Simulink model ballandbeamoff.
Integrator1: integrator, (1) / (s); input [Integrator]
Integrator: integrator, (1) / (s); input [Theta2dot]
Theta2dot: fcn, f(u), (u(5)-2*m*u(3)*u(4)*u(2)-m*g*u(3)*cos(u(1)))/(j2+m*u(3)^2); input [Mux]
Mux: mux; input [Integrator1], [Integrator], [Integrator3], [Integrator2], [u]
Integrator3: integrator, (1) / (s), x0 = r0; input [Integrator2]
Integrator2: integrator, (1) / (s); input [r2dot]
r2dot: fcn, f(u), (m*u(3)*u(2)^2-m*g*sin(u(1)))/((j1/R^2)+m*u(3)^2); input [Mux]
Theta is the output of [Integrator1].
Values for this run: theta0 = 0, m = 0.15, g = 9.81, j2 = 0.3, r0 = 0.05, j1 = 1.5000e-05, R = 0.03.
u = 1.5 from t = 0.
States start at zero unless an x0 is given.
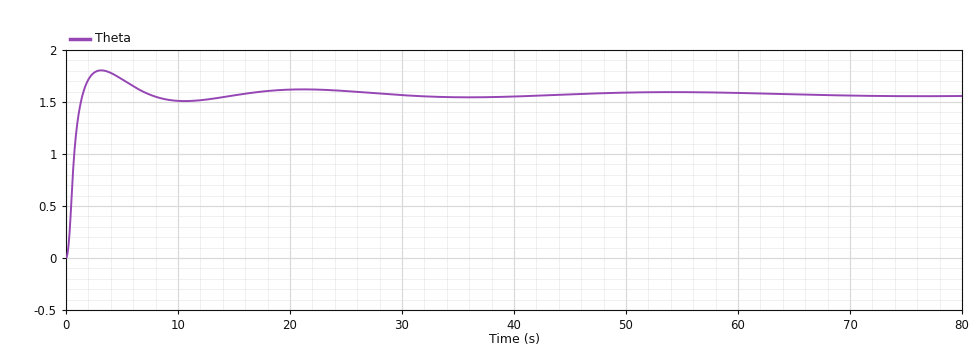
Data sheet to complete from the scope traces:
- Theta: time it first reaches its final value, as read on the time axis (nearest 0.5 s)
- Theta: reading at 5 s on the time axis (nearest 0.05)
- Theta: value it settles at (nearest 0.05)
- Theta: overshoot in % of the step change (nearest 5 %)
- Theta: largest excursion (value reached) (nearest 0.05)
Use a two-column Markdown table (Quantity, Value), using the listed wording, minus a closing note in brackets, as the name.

| Quantity | Value |
|---|---|
| Theta: time it first reaches its final value, as read on the time axis | 1.5 s |
| Theta: reading at 5 s on the time axis | 1.70 |
| Theta: value it settles at | 1.55 |
| Theta: overshoot in % of the step change | 15 % |
| Theta: largest excursion (value reached) | 1.80 |
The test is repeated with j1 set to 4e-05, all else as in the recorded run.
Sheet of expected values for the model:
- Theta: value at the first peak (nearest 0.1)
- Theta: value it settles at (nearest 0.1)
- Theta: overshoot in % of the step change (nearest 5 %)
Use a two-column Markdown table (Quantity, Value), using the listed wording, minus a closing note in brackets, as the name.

| Quantity | Value |
|---|---|
| Theta: value at the first peak | 1.9 |
| Theta: value it settles at | 1.6 |
| Theta: overshoot in % of the step change | 20 % |
